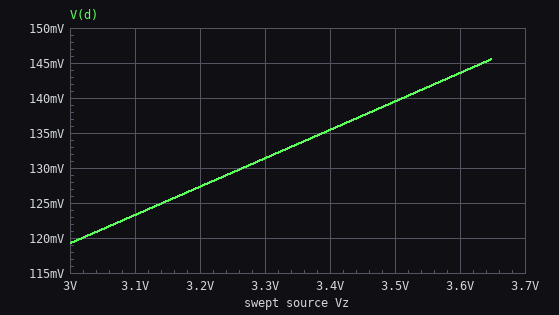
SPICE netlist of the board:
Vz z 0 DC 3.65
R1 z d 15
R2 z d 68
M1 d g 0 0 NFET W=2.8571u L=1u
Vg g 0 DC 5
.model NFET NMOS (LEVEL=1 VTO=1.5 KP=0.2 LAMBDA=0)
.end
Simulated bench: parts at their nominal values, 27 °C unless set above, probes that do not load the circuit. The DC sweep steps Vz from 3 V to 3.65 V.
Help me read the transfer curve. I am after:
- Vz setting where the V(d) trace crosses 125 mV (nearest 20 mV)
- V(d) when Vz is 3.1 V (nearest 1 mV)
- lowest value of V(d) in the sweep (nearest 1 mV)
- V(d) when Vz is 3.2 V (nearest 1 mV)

3.14 V
123 mV
119 mV
127 mV
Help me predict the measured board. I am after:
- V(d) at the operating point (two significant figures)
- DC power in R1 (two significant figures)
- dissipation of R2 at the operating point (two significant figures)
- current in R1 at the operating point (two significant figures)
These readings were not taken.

150 mV
820 mW
180 mW
230 mA
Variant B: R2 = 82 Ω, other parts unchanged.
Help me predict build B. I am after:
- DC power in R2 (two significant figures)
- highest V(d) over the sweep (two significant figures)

150 mW
140 mV
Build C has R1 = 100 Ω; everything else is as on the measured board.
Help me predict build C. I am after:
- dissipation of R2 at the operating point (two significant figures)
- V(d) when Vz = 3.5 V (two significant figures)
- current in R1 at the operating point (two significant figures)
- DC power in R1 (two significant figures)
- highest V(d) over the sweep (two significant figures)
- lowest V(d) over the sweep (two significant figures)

190 mW
43 mV
36 mA
130 mW
45 mV
37 mV
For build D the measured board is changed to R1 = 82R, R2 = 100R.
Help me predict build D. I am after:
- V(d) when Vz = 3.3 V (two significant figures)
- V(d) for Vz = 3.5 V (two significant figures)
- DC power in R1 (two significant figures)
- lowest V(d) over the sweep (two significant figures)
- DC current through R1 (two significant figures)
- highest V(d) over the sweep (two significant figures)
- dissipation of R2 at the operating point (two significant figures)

36 mV
39 mV
160 mW
33 mV
44 mA
40 mV
130 mW
